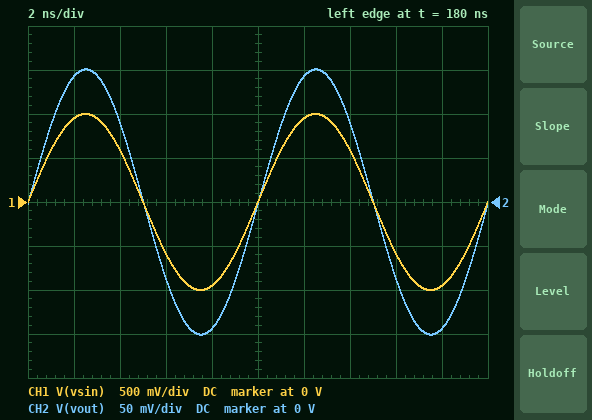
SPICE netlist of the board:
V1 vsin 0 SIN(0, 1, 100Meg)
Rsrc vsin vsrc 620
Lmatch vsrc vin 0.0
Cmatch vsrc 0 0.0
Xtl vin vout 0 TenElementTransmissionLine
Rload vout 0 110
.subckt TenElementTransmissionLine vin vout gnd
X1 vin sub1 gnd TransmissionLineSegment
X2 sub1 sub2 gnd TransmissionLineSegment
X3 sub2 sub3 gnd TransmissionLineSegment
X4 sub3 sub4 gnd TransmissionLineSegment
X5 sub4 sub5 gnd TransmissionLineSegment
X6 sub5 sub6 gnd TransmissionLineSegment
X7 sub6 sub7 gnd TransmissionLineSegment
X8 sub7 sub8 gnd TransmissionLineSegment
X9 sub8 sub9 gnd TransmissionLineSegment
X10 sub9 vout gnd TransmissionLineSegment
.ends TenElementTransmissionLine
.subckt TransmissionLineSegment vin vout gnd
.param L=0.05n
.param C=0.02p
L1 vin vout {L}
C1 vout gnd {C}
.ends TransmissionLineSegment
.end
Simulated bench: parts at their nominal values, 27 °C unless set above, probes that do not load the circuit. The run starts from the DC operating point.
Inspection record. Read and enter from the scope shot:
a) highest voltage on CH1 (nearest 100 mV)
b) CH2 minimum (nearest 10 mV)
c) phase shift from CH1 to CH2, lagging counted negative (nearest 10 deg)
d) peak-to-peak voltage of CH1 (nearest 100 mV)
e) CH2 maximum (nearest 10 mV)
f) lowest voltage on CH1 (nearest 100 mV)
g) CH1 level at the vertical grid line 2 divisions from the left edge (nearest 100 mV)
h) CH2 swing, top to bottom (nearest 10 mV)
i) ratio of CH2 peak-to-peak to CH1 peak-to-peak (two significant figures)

1.0 V
-150 mV
0 deg
2.0 V
150 mV
-1.0 V
600 mV
300 mV
0.15
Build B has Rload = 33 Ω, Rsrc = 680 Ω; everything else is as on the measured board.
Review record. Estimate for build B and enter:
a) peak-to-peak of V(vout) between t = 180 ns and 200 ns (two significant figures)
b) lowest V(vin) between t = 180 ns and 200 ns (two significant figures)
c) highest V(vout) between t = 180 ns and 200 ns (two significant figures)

93 mV
-46 mV
46 mV
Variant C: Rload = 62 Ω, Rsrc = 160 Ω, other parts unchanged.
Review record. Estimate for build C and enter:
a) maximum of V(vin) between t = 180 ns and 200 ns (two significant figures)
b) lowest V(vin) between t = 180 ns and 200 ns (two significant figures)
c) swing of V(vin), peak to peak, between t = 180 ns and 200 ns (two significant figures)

280 mV
-280 mV
560 mV
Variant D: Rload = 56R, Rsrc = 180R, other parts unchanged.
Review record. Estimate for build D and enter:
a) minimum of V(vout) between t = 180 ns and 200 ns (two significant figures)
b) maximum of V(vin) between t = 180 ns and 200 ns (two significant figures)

-240 mV
240 mV
